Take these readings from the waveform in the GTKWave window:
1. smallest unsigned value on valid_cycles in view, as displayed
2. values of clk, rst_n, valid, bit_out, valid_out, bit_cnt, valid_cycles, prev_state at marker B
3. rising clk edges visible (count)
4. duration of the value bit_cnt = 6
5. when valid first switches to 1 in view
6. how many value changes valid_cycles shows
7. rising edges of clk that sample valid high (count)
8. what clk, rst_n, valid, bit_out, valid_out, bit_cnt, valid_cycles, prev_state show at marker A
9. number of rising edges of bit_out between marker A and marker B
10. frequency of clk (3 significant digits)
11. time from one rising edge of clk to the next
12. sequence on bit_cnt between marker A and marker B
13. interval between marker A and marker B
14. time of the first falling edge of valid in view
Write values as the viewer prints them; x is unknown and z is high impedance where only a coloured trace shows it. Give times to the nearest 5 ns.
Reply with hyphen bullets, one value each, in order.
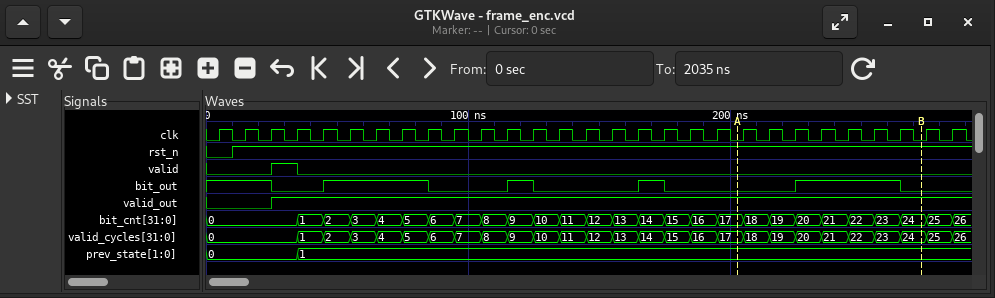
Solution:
- 0
- clk=0, rst_n=1, valid=0, bit_out=0, valid_out=1, bit_cnt=24, valid_cycles=24, prev_state=1
- 29
- 10 ns
- 25 ns
- 26
- 1
- clk=0, rst_n=1, valid=0, bit_out=0, valid_out=1, bit_cnt=17, valid_cycles=17, prev_state=1
- 1
- 100 MHz
- 10 ns
- 17, 18, 19, 20, 21, 22, 23, 24
- 70 ns
- 35 ns
